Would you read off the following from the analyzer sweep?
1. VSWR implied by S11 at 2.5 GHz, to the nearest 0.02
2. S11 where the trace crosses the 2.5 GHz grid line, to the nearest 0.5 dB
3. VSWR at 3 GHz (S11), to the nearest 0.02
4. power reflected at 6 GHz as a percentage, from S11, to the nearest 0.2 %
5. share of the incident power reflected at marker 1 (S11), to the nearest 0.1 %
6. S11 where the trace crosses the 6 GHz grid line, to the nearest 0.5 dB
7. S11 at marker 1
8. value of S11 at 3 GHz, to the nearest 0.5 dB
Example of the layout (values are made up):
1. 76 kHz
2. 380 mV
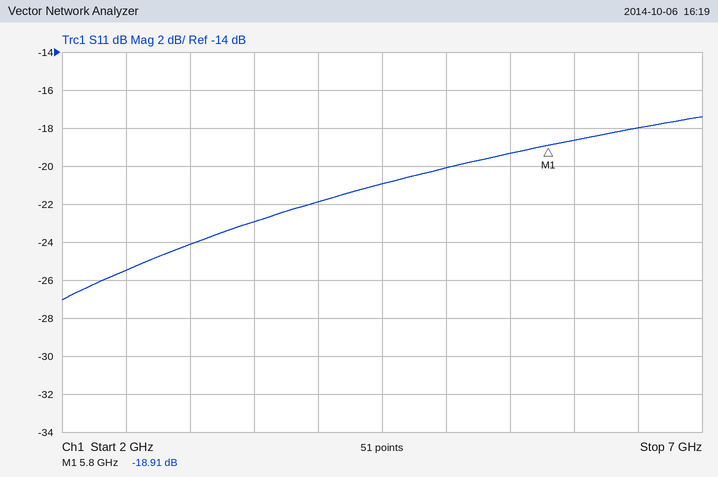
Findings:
1. 1.12
2. -25.5 dB
3. 1.14
4. 1.4 %
5. 1.3 %
6. -18.5 dB
7. -18.91 dB
8. -24.0 dB
